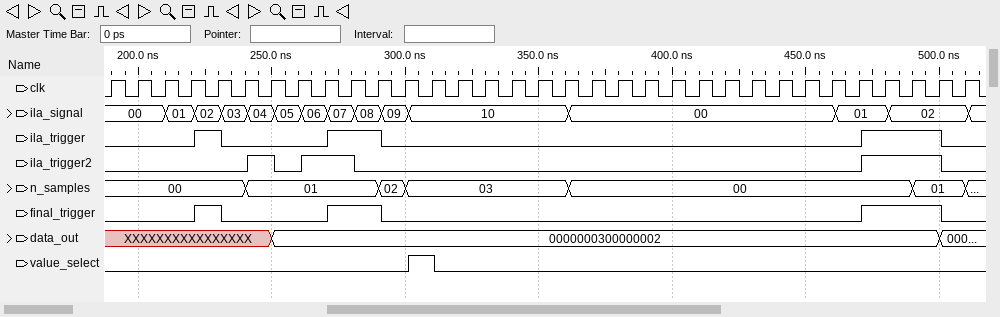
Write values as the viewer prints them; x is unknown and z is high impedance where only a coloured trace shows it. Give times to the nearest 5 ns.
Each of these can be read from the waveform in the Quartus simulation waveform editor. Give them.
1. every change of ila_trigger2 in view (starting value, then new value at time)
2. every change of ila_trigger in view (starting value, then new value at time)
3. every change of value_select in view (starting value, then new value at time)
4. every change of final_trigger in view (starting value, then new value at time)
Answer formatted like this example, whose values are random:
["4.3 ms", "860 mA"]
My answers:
["0, 1 at 240 ns, 0 at 250 ns, 1 at 260 ns, 0 at 280 ns, 1 at 470 ns, 0 at 500 ns", "0, 1 at 220 ns, 0 at 230 ns, 1 at 270 ns, 0 at 290 ns, 1 at 470 ns, 0 at 500 ns", "0, 1 at 300 ns, 0 at 310 ns", "0, 1 at 220 ns, 0 at 230 ns, 1 at 270 ns, 0 at 290 ns, 1 at 470 ns, 0 at 500 ns"]
